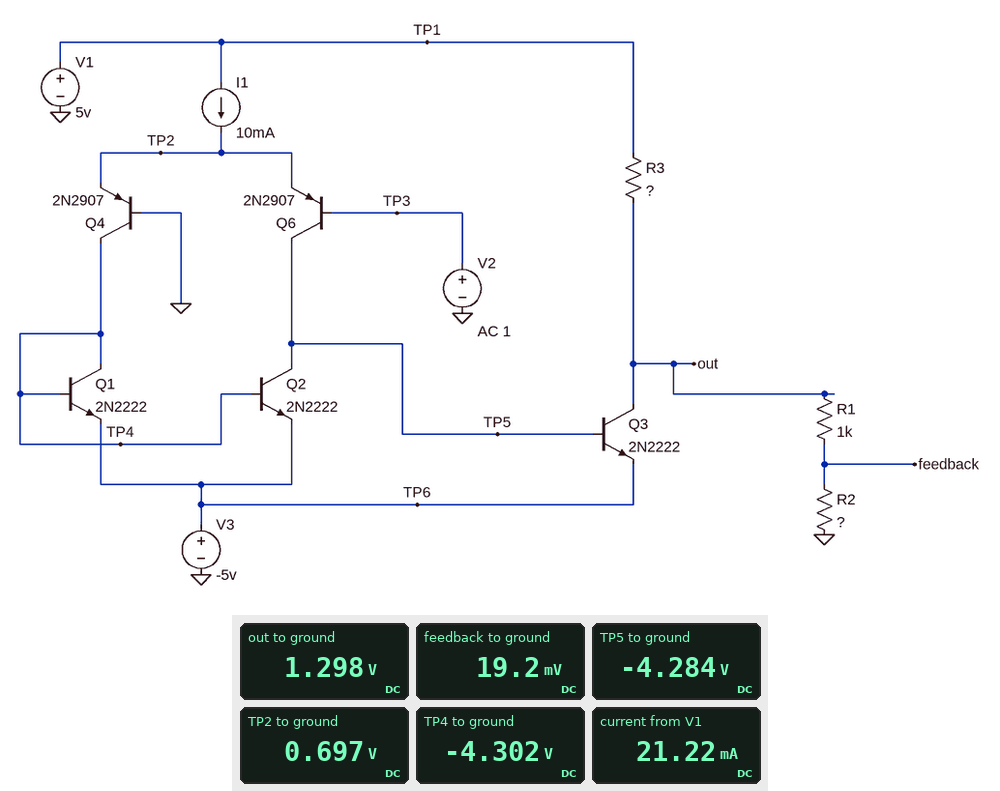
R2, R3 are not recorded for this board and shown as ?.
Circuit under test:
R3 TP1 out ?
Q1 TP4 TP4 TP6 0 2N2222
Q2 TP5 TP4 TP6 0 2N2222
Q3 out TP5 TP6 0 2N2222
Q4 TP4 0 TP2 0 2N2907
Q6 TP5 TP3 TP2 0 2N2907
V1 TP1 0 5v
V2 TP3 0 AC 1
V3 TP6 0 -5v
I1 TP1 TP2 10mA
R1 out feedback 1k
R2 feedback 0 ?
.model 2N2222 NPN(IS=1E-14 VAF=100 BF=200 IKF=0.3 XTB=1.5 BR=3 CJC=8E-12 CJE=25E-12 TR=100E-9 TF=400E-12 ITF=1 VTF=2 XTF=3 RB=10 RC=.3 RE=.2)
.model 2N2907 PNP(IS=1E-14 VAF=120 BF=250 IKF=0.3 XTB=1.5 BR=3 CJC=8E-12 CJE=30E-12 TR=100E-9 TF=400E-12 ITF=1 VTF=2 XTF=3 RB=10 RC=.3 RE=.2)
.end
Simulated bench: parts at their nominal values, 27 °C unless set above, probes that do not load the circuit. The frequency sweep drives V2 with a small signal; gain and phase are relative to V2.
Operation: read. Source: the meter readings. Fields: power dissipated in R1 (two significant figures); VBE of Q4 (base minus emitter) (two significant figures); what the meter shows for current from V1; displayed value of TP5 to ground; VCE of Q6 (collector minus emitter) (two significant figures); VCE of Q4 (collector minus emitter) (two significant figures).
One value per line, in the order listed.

1.6 mW
-700 mV
21.22 mA
-4.284 V
-5.0 V
-5.0 V
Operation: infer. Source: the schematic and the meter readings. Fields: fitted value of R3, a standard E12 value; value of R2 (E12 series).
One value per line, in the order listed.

330 Ω
15 Ω
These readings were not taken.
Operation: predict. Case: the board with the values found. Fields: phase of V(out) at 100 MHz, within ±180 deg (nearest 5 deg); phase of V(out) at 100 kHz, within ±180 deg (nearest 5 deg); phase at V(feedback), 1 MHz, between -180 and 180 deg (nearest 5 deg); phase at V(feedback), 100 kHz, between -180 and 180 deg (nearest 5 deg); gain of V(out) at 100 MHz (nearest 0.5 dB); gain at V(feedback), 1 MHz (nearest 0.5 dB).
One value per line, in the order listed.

-165 deg
-10 deg
-65 deg
-10 deg
28.0 dB
35.0 dB
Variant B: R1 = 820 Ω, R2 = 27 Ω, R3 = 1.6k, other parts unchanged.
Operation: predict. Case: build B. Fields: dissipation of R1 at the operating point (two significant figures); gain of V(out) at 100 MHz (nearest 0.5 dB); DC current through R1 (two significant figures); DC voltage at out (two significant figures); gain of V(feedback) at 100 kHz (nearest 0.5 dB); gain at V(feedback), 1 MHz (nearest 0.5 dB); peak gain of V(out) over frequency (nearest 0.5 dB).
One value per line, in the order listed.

14 mW
26.5 dB
4.2 mA
-3.5 V
54.0 dB
41.5 dB
84.5 dB
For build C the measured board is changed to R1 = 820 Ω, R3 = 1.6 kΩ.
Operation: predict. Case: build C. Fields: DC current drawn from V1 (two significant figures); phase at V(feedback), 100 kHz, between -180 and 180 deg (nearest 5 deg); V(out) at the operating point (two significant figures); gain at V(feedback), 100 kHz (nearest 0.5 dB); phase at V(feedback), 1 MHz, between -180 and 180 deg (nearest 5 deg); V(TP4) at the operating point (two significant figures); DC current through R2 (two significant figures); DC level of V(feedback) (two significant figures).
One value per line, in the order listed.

15 mA
-25 deg
-3.5 V
49.0 dB
-80 deg
-4.3 V
4.2 mA
-63 mV
